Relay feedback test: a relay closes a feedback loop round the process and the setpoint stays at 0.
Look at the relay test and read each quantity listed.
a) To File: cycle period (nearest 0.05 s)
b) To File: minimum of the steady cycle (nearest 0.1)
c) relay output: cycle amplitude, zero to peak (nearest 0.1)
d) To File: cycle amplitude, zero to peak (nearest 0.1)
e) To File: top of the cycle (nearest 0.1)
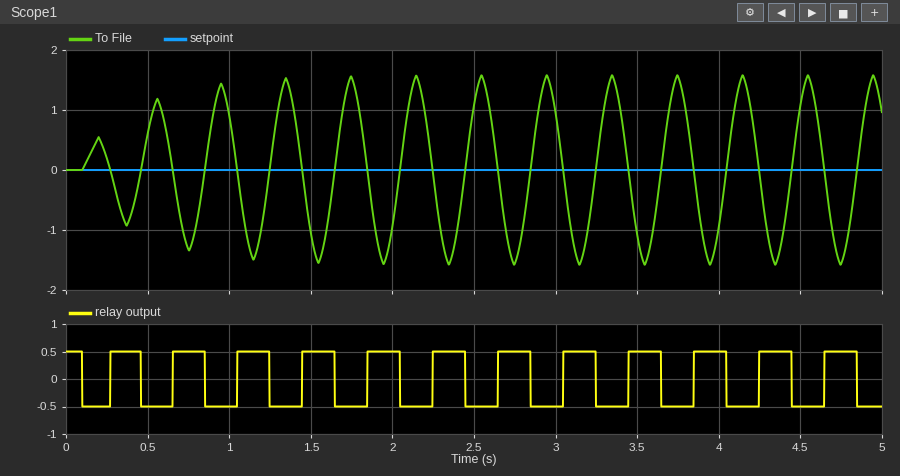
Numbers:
0.40 s
-1.6
0.5
1.6
1.6
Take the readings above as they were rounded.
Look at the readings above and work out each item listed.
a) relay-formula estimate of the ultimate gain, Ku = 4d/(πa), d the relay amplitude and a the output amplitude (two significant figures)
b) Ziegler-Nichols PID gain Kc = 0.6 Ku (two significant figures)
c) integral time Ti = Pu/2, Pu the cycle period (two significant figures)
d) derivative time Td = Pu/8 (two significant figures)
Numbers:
0.40
0.24
0.20 s
0.050 s
